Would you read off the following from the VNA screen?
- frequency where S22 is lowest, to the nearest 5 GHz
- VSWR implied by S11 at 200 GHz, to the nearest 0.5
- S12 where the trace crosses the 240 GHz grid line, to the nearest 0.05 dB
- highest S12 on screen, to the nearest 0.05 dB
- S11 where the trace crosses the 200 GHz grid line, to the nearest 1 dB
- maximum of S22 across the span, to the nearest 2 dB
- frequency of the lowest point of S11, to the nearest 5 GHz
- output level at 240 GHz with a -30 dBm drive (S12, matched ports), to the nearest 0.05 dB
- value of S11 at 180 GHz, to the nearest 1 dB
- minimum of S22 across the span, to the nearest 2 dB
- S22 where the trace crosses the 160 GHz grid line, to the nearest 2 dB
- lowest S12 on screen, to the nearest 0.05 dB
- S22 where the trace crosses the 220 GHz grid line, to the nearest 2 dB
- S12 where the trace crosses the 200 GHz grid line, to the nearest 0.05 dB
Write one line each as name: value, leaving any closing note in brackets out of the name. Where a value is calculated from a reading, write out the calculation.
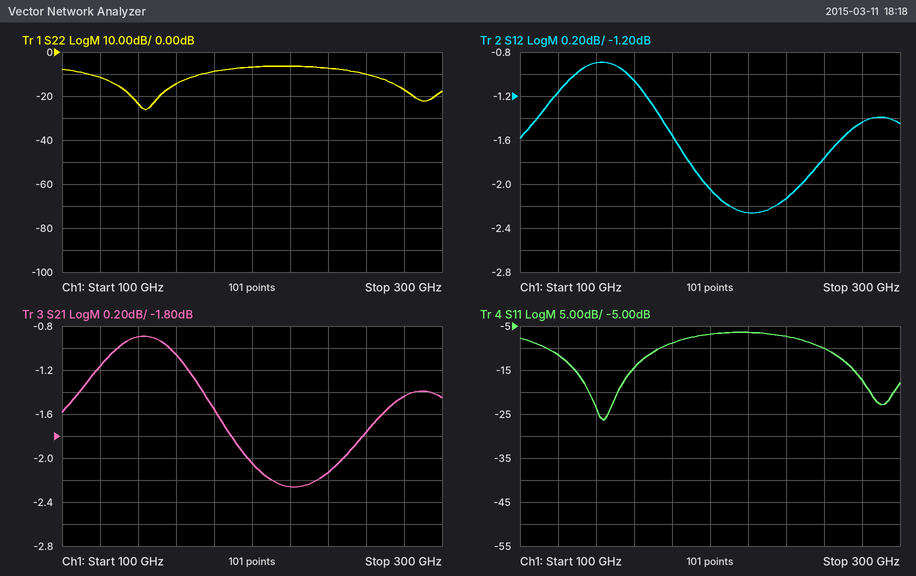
frequency where S22 is lowest, to the nearest 5 GHz: 145 GHz
VSWR implied by S11 at 200 GHz, to the nearest 0.5: |Γ| = 10^(-7/20) = 0.4467; VSWR = (1 + 0.4467)/(1 − 0.4467) ≈ 2.61, so 2.5 to the nearest 0.5
S12 where the trace crosses the 240 GHz grid line, to the nearest 0.05 dB: -2.15 dB
highest S12 on screen, to the nearest 0.05 dB: -0.90 dB
S11 where the trace crosses the 200 GHz grid line, to the nearest 1 dB: -7 dB
maximum of S22 across the span, to the nearest 2 dB: -6 dB
frequency of the lowest point of S11, to the nearest 5 GHz: 145 GHz
output level at 240 GHz with a -30 dBm drive (S12, matched ports), to the nearest 0.05 dB: -30 dBm + (-2.15 dB) = -32.15 dBm
value of S11 at 180 GHz, to the nearest 1 dB: -9 dB
minimum of S22 across the span, to the nearest 2 dB: -26 dB
S22 where the trace crosses the 160 GHz grid line, to the nearest 2 dB: -14 dB
lowest S12 on screen, to the nearest 0.05 dB: -2.25 dB
S22 where the trace crosses the 220 GHz grid line, to the nearest 2 dB: -6 dB
S12 where the trace crosses the 200 GHz grid line, to the nearest 0.05 dB: -2.05 dB
